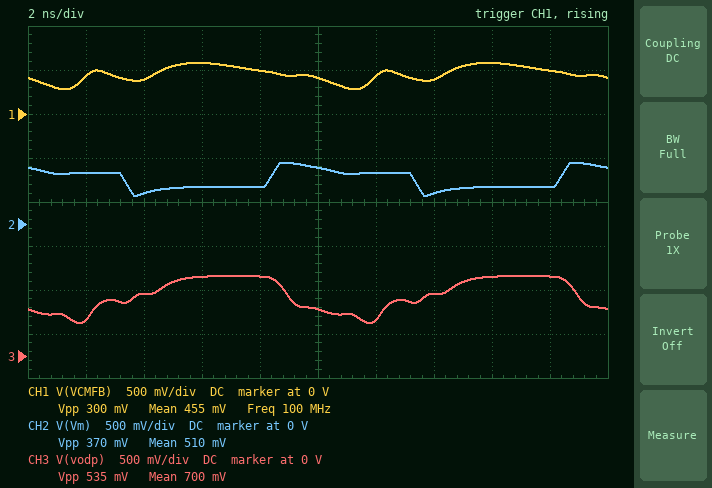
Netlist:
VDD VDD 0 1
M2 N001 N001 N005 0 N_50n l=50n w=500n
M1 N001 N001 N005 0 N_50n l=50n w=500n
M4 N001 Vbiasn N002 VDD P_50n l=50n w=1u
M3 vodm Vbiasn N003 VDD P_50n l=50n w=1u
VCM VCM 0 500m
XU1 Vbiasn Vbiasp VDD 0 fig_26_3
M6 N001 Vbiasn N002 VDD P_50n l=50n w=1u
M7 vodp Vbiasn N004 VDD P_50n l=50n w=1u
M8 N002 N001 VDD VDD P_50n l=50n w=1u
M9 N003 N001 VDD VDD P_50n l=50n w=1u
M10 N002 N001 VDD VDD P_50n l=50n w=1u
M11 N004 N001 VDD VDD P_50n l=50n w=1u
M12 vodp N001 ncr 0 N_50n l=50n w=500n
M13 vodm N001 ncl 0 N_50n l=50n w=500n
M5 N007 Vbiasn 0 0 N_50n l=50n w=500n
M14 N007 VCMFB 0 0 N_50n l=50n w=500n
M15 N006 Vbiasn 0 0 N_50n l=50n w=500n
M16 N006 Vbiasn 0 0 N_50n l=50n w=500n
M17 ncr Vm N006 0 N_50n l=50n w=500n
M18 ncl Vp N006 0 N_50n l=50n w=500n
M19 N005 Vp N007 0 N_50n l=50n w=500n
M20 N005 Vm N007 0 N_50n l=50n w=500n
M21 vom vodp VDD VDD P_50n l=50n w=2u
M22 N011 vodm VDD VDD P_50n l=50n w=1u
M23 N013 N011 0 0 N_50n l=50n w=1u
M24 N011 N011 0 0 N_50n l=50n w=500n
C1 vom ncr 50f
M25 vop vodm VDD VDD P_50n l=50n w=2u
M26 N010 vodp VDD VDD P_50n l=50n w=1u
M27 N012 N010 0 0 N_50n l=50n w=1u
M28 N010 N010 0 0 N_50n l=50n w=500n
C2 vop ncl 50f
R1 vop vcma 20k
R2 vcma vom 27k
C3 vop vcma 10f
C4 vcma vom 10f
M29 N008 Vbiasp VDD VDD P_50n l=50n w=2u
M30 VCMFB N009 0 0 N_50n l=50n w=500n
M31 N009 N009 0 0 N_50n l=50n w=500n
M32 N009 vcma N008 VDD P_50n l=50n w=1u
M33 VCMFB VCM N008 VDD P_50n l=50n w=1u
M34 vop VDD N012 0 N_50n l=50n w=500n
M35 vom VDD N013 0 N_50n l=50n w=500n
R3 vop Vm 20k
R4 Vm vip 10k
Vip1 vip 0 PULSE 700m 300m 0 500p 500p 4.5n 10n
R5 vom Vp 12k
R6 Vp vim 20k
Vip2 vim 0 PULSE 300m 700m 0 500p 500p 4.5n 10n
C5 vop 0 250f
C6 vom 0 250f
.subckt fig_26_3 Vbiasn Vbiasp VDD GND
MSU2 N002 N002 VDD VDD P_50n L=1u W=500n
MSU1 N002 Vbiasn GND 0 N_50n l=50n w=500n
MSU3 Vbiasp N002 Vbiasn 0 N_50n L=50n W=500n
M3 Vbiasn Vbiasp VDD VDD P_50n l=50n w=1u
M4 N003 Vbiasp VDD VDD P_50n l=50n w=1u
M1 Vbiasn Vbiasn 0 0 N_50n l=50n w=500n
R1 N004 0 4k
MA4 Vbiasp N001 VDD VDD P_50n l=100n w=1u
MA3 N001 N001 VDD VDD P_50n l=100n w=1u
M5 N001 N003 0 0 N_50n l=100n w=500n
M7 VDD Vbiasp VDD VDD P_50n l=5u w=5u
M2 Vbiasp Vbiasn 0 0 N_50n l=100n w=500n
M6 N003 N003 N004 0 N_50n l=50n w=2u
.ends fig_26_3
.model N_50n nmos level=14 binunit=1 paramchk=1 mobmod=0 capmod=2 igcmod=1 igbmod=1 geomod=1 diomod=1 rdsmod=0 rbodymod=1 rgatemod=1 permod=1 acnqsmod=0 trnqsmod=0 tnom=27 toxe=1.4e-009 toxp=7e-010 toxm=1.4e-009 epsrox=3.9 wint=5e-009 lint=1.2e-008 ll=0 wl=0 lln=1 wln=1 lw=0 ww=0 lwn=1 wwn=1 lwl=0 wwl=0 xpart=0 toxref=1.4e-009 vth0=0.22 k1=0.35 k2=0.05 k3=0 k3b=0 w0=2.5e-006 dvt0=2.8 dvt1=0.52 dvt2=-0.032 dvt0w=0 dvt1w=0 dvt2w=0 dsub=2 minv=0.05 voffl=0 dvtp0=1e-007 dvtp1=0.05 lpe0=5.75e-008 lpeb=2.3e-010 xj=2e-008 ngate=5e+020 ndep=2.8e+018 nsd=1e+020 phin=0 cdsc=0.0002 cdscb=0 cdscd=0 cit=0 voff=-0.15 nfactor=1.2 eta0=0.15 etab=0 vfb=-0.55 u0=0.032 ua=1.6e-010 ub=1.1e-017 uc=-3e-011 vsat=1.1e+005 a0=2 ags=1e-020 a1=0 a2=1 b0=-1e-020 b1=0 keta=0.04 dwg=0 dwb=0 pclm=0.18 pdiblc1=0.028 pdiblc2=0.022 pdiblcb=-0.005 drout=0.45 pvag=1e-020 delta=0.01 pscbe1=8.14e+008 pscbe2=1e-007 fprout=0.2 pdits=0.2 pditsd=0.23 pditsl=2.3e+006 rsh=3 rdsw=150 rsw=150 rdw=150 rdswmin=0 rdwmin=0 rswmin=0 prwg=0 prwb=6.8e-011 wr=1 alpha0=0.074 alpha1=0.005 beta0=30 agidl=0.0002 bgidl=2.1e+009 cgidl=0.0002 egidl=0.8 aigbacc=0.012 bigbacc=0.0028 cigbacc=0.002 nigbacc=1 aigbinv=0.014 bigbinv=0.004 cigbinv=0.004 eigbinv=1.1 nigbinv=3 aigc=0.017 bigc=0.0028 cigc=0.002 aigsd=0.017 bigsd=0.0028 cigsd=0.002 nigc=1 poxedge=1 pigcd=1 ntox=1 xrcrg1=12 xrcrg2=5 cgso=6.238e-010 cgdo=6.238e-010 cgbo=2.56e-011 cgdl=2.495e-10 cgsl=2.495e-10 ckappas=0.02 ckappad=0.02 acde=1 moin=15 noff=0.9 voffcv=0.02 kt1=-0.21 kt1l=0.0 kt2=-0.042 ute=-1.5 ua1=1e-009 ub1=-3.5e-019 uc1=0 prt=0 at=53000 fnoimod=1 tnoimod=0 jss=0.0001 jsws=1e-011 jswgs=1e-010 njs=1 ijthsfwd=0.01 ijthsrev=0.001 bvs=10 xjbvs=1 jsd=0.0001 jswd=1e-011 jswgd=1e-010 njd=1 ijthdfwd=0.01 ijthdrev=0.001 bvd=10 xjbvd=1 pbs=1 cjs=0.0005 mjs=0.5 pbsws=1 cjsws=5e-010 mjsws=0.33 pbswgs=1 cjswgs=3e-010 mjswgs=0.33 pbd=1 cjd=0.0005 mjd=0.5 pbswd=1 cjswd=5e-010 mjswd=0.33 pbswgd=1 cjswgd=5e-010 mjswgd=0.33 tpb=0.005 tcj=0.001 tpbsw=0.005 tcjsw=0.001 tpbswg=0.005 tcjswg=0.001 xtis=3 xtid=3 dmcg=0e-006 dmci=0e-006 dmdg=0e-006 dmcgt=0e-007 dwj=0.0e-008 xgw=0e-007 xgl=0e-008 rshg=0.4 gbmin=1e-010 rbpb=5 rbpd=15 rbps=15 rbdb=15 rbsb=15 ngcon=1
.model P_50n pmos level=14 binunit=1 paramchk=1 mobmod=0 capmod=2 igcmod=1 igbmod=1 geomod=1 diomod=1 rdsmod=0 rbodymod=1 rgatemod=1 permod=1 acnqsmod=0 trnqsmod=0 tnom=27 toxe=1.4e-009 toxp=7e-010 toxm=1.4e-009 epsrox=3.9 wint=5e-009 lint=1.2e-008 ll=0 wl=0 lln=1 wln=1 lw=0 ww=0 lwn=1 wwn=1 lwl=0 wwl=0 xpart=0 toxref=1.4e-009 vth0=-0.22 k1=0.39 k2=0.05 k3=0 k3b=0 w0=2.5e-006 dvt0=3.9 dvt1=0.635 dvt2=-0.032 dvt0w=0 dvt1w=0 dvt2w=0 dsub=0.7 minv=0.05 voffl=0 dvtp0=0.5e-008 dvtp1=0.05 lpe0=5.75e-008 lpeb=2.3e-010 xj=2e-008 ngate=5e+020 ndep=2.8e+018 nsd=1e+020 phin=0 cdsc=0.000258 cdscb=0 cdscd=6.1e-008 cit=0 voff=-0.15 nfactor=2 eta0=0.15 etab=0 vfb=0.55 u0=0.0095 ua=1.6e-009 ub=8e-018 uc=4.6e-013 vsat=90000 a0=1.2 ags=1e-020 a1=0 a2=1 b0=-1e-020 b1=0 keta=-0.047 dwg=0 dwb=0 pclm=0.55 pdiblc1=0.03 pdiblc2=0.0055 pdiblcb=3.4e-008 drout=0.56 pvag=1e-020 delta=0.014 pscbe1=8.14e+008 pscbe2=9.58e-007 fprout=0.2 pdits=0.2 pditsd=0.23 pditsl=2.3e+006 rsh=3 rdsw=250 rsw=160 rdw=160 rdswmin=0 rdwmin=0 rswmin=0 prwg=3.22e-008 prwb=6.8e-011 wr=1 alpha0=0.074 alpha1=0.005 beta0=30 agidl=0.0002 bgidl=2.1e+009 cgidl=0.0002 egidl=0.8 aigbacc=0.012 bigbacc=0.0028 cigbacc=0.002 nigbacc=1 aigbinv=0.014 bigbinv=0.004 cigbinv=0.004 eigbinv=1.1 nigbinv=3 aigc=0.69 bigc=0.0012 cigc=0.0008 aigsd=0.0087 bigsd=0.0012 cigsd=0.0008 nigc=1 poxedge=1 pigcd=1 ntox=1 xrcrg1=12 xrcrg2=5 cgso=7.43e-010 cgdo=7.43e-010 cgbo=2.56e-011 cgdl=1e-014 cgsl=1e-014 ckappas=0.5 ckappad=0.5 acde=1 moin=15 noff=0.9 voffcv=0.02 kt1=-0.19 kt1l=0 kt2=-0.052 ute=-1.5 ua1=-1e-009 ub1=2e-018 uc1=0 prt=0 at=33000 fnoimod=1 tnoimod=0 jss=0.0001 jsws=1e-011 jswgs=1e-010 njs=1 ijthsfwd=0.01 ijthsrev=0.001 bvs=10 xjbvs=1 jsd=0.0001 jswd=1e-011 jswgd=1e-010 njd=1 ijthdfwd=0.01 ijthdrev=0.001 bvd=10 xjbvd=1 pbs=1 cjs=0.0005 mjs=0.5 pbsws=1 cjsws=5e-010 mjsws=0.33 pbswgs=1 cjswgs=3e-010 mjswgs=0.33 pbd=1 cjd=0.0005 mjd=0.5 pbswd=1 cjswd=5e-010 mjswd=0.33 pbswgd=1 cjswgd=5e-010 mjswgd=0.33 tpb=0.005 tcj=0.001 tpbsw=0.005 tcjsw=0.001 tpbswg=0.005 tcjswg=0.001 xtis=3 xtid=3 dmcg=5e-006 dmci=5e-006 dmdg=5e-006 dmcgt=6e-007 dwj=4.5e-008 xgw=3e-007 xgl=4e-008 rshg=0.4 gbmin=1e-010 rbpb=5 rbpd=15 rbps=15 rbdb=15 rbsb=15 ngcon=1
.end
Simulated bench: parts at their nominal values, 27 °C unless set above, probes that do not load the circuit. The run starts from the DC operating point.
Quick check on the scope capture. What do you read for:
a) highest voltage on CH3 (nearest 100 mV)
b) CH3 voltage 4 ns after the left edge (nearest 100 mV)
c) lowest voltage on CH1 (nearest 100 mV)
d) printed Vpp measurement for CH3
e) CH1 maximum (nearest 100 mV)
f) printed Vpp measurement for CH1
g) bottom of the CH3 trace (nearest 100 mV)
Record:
900 mV
700 mV
300 mV
535 mV
600 mV
300 mV
400 mV
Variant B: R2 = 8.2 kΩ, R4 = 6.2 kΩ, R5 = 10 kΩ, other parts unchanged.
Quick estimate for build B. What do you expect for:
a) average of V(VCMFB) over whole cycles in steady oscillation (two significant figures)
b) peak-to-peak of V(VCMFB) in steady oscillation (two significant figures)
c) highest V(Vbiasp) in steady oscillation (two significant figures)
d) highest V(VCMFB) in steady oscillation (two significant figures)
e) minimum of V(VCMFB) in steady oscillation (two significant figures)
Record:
580 mV
810 mV
590 mV
870 mV
58 mV
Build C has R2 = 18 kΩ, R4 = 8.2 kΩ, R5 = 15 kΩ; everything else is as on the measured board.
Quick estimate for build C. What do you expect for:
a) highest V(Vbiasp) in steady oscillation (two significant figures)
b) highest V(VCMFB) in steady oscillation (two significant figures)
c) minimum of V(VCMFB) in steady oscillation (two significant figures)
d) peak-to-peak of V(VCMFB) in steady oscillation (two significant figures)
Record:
590 mV
460 mV
350 mV
110 mV
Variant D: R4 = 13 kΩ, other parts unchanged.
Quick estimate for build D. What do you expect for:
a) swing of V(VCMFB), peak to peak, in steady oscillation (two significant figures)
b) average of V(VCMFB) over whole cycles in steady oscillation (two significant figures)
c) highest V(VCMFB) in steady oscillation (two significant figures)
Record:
290 mV
450 mV
560 mV
